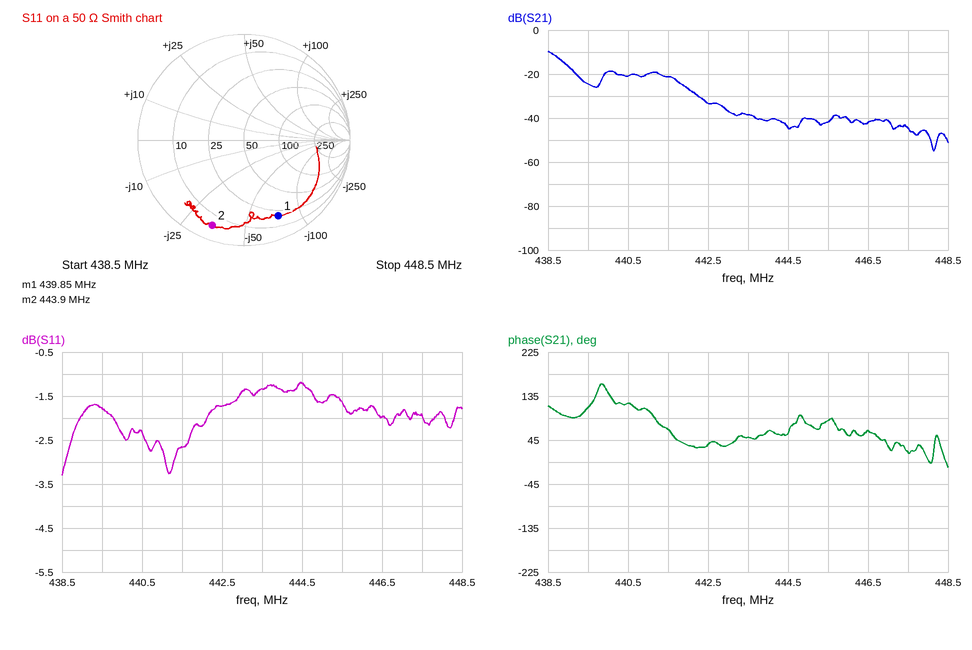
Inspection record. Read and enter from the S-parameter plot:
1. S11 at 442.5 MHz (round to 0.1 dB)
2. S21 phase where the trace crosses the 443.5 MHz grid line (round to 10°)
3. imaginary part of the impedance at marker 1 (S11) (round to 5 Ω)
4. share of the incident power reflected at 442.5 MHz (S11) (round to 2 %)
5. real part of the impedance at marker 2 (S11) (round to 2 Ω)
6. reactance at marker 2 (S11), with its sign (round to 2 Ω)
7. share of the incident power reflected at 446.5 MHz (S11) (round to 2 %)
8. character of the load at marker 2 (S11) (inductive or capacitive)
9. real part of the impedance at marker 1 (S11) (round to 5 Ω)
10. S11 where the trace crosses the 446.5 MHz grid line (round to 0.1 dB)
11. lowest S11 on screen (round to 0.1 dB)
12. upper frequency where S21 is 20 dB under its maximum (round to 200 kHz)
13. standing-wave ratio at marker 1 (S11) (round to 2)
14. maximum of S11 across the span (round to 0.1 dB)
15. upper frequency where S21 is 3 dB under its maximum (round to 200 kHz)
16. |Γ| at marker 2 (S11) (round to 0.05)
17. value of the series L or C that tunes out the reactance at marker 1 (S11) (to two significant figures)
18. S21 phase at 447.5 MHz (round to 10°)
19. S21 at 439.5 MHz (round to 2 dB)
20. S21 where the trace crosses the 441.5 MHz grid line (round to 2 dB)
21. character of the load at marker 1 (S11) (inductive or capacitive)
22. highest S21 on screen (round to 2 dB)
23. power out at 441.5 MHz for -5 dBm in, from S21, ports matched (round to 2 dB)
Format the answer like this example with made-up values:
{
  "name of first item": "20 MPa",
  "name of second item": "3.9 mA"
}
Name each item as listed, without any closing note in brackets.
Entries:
{
  "S11 at 442.5 MHz": "-1.7 dB",
  "S21 phase where the trace crosses the 443.5 MHz grid line": "50°",
  "imaginary part of the impedance at marker 1 (S11)": "-75 Ω",
  "share of the incident power reflected at 442.5 MHz (S11)": "68 %",
  "real part of the impedance at marker 2 (S11)": "6 Ω",
  "reactance at marker 2 (S11), with its sign": "-34 Ω",
  "share of the incident power reflected at 446.5 MHz (S11)": "64 %",
  "character of the load at marker 2 (S11)": "capacitive",
  "real part of the impedance at marker 1 (S11)": "20 Ω",
  "S11 where the trace crosses the 446.5 MHz grid line": "-2.0 dB",
  "lowest S11 on screen": "-3.3 dB",
  "upper frequency where S21 is 20 dB under its maximum": "442.2 MHz",
  "standing-wave ratio at marker 1 (S11)": "8",
  "maximum of S11 across the span": "-1.2 dB",
  "upper frequency where S21 is 3 dB under its maximum": "438.8 MHz",
  "|Γ| at marker 2 (S11)": "0.85",
  "value of the series L or C that tunes out the reactance at marker 1 (S11)": "27 nH",
  "S21 phase at 447.5 MHz": "20°",
  "S21 at 439.5 MHz": "-24 dB",
  "S21 where the trace crosses the 441.5 MHz grid line": "-22 dB",
  "character of the load at marker 1 (S11)": "capacitive",
  "highest S21 on screen": "-10 dB",
  "power out at 441.5 MHz for -5 dBm in, from S21, ports matched": "-26 dBm"
}
